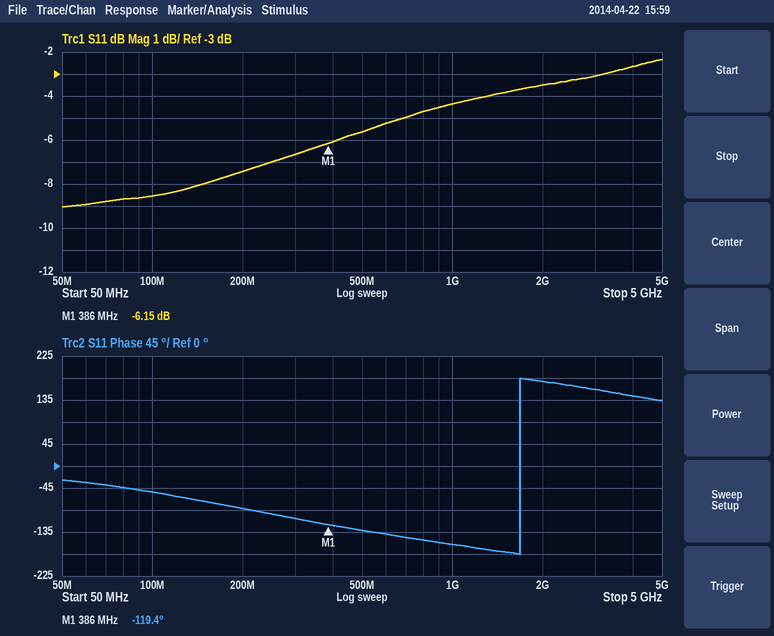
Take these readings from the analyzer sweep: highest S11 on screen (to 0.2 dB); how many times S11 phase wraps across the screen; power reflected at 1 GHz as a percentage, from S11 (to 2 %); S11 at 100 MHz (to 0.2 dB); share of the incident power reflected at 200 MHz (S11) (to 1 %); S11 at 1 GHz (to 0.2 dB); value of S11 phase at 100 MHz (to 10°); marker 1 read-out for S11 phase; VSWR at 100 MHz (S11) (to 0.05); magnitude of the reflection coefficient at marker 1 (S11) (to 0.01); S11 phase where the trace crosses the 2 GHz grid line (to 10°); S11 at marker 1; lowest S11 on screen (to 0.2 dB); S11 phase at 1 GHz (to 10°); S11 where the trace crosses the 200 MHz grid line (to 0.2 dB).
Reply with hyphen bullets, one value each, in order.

- -2.4 dB
- 1
- 36 %
- -8.6 dB
- 18 %
- -4.4 dB
- -50°
- -119.4°
- 2.20
- 0.49
- 170°
- -6.15 dB
- -9.0 dB
- -160°
- -7.4 dB
